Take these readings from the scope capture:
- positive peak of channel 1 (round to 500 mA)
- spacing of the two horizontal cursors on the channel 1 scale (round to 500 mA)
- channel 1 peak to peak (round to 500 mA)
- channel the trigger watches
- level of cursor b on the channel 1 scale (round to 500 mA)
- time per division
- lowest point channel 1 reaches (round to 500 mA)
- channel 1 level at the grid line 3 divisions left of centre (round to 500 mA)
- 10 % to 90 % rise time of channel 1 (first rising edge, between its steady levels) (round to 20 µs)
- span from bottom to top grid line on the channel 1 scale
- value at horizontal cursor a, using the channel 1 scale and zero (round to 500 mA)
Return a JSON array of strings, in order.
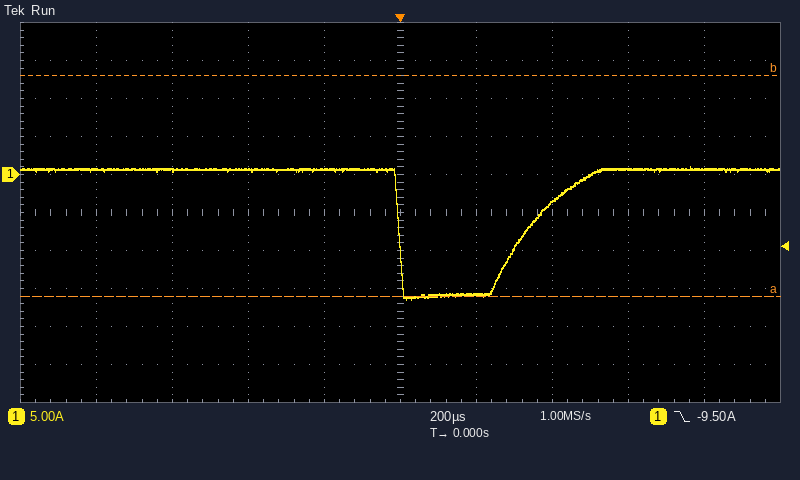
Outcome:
["1.0 A", "29.0 A", "17.5 A", "channel 1", "13.0 A", "200 µs", "-16.5 A", "500 mA", "220 µs", "50 A", "-16.0 A"]
